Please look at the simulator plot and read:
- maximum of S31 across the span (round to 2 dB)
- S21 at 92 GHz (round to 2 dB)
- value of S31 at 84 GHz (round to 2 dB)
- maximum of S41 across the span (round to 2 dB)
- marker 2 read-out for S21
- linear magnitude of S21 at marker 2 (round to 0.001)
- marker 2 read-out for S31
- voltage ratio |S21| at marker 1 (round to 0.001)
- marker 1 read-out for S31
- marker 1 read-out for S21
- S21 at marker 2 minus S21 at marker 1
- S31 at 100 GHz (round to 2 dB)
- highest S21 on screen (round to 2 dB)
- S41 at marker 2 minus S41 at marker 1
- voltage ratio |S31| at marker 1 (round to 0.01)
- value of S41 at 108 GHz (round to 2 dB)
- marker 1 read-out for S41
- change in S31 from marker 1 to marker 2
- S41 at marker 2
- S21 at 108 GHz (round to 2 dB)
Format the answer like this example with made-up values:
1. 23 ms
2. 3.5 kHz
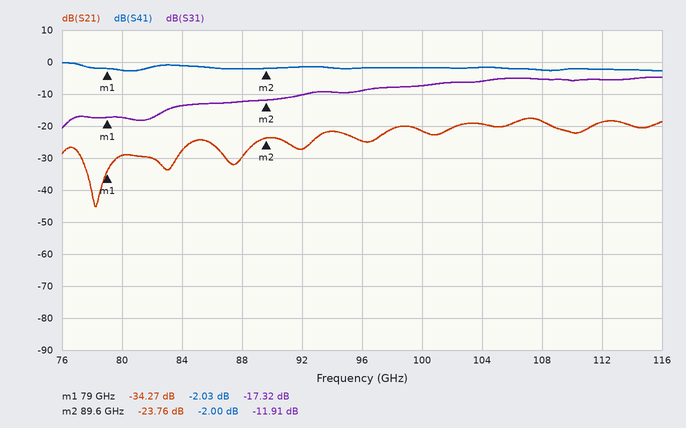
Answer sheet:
1. -4 dB
2. -28 dB
3. -14 dB
4. 0 dB
5. -23.76 dB
6. 0.065
7. -11.91 dB
8. 0.019
9. -17.32 dB
10. -34.27 dB
11. 10.51 dB
12. -8 dB
13. -18 dB
14. 0.03 dB
15. 0.14
16. -2 dB
17. -2.03 dB
18. 5.41 dB
19. -2.00 dB
20. -18 dB
